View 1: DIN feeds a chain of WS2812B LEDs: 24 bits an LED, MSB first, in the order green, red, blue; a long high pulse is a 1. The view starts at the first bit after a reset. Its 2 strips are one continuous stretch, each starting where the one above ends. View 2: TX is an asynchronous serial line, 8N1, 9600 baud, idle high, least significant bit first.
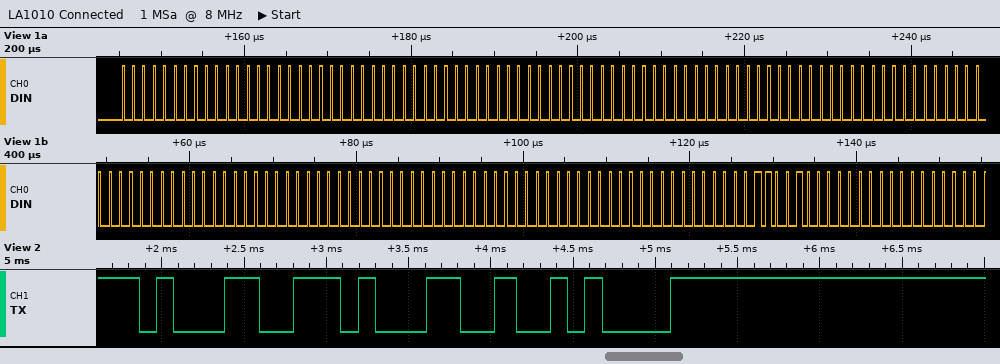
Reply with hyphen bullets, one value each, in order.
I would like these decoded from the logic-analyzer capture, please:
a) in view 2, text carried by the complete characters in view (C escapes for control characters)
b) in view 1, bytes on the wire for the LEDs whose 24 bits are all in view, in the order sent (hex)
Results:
- "11\n"
- 00 00 00 00 00 00 00 00 00 00 00 00 00 00 00 00 00 00 32 00 00
